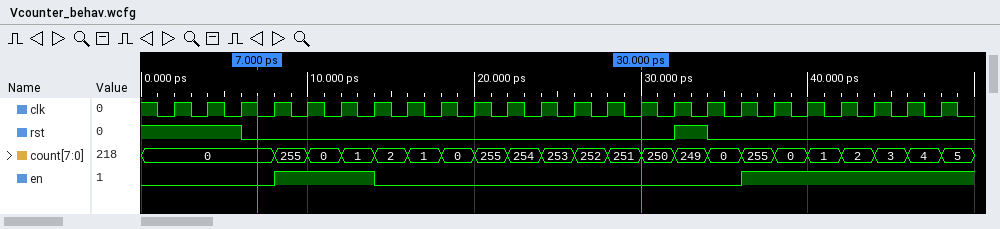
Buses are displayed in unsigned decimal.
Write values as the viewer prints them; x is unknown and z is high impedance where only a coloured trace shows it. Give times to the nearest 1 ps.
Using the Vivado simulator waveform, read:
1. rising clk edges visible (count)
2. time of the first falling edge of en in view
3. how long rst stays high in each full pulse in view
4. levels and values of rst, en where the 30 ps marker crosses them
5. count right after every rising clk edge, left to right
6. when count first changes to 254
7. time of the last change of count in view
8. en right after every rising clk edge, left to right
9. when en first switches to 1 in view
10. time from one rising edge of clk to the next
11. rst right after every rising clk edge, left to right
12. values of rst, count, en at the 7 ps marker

24
14 ps
2 ps
rst=0, en=0
0, 0, 0, 255, 0, 1, 2, 1, 0, 255, 254, 253, 252, 251, 250, 249, 0, 255, 0, 1, 2, 3, 4, 5
22 ps
48 ps
0 0 0 1 1 1 0 0 0 0 0 0 0 0 0 0 0 1 1 1 1 1 1 1
8 ps
2 ps
1 1 0 0 0 0 0 0 0 0 0 0 0 0 0 1 0 0 0 0 0 0 0 0
rst=0, count=0, en=0
